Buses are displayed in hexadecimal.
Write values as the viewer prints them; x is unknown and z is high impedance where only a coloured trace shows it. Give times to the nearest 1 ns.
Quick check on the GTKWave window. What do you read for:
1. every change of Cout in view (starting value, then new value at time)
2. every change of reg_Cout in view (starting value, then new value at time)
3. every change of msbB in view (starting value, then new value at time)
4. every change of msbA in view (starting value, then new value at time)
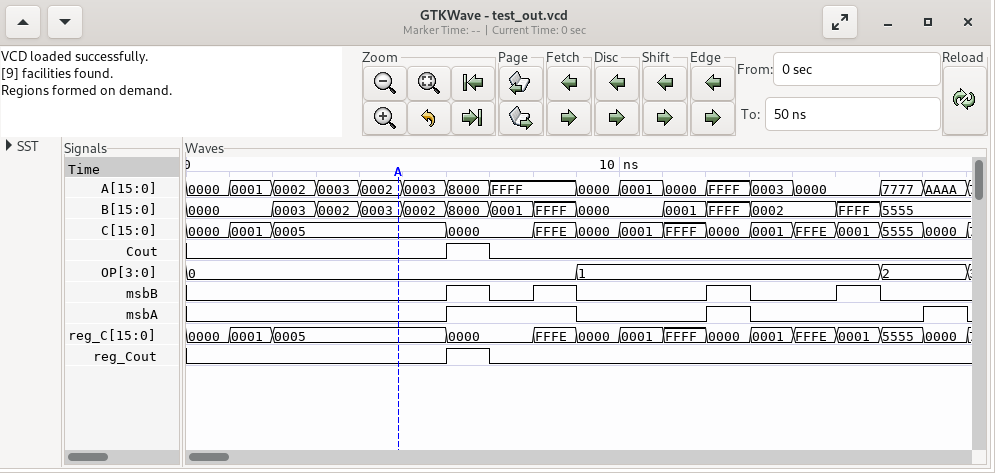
0, 1 at 6 ns, 0 at 7 ns
0, 1 at 6 ns, 0 at 7 ns
0, 1 at 6 ns, 0 at 7 ns, 1 at 8 ns, 0 at 9 ns, 1 at 12 ns, 0 at 13 ns, 1 at 15 ns, 0 at 16 ns
0, 1 at 6 ns, 0 at 9 ns, 1 at 12 ns, 0 at 13 ns, 1 at 17 ns, 0 at 18 ns
